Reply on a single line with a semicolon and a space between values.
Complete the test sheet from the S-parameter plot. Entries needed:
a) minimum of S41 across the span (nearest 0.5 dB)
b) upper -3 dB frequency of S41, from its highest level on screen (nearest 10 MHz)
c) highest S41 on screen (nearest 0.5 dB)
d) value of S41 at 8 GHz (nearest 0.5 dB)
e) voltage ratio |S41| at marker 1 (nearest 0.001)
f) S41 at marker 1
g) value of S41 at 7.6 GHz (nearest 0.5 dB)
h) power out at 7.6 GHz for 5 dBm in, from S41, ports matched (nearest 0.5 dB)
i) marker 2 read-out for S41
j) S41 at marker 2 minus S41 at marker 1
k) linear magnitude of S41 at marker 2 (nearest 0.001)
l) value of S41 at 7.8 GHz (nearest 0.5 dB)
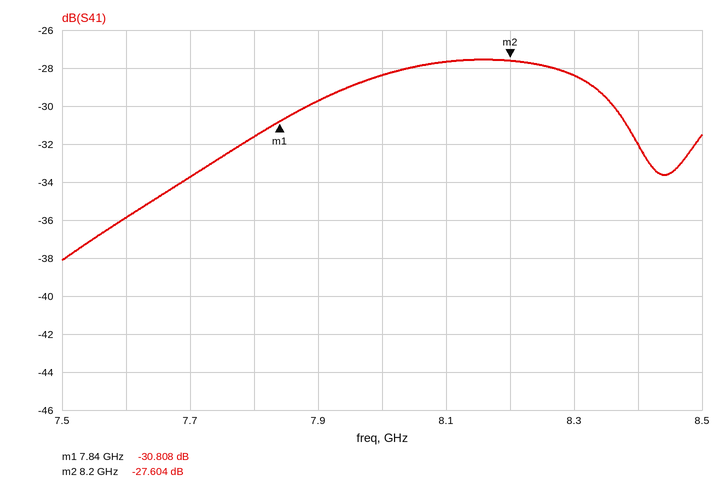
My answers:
-38.0 dB; 8.37 GHz; -27.5 dB; -28.5 dB; 0.029; -30.808 dB; -36.0 dB; -31.0 dBm; -27.604 dB; 3.204 dB; 0.042; -31.5 dB
